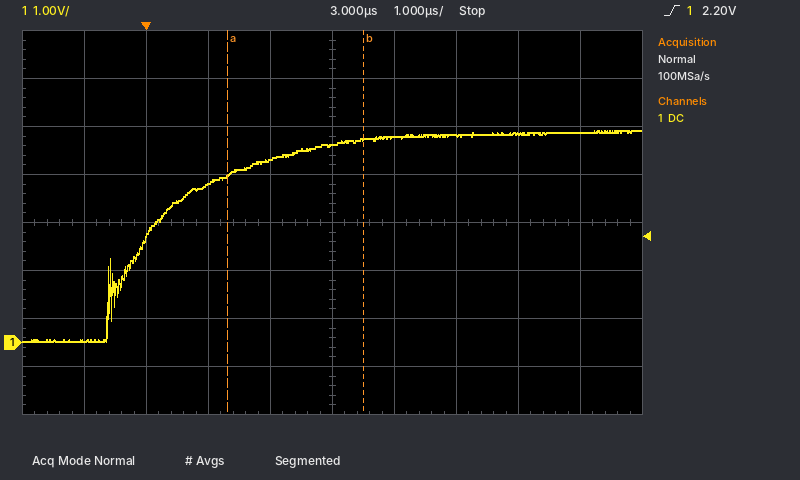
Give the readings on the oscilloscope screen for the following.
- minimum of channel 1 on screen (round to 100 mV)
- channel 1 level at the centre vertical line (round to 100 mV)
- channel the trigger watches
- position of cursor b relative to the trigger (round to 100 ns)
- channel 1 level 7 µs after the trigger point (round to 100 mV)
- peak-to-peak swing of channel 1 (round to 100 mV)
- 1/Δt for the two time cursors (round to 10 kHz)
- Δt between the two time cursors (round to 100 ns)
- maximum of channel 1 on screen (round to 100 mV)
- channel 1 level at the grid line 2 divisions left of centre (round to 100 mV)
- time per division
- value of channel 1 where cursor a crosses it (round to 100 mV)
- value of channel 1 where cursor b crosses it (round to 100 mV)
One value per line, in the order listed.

0.0 V
4.1 V
channel 1
+3.5 µs
4.4 V
4.4 V
450 kHz
2.2 µs
4.4 V
3.3 V
1 µs
3.5 V
4.2 V
